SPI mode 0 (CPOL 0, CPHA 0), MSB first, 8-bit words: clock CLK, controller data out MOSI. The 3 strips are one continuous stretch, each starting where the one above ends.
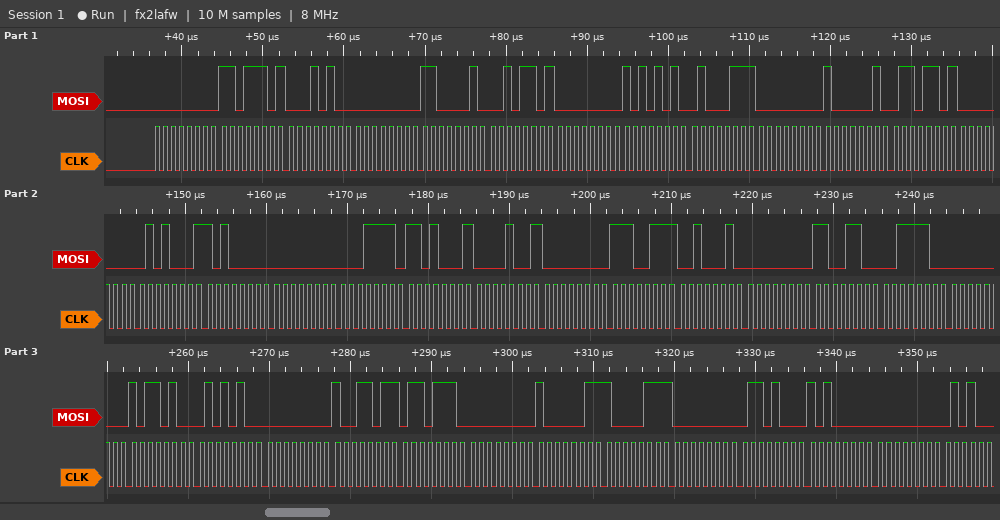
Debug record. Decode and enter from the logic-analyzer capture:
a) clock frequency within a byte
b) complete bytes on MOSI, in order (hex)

1 MHz
0x00 0xDD 0x14 0x00 0xC2 0x2D 0x00 0xAA 0x47 0x00 0x82 0x6D 0x00 0x51 0xA0 0x00 0x1E 0xD1 0x09 0x00 0xE7 0x22 0x00 0xCC 0x3C 0x00 0xB4 0x54 0x00 0x9B 0x6E 0x00 0x83 0x87 0x00 0x68 0xA0 0x00
